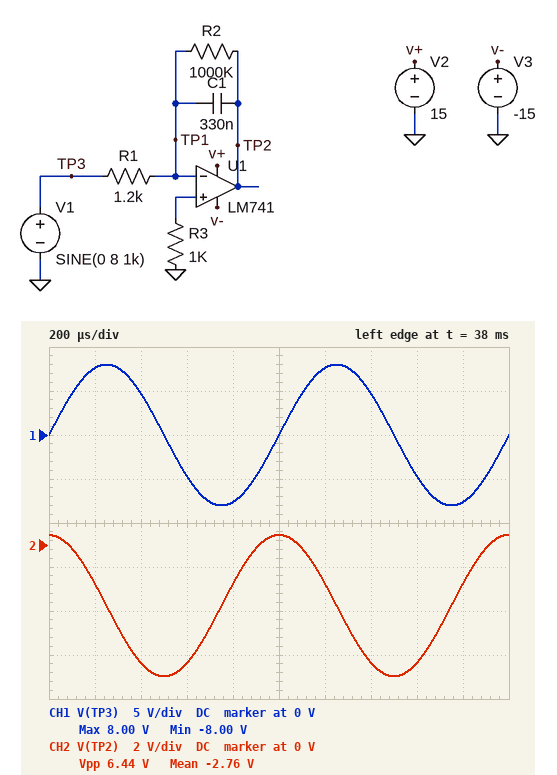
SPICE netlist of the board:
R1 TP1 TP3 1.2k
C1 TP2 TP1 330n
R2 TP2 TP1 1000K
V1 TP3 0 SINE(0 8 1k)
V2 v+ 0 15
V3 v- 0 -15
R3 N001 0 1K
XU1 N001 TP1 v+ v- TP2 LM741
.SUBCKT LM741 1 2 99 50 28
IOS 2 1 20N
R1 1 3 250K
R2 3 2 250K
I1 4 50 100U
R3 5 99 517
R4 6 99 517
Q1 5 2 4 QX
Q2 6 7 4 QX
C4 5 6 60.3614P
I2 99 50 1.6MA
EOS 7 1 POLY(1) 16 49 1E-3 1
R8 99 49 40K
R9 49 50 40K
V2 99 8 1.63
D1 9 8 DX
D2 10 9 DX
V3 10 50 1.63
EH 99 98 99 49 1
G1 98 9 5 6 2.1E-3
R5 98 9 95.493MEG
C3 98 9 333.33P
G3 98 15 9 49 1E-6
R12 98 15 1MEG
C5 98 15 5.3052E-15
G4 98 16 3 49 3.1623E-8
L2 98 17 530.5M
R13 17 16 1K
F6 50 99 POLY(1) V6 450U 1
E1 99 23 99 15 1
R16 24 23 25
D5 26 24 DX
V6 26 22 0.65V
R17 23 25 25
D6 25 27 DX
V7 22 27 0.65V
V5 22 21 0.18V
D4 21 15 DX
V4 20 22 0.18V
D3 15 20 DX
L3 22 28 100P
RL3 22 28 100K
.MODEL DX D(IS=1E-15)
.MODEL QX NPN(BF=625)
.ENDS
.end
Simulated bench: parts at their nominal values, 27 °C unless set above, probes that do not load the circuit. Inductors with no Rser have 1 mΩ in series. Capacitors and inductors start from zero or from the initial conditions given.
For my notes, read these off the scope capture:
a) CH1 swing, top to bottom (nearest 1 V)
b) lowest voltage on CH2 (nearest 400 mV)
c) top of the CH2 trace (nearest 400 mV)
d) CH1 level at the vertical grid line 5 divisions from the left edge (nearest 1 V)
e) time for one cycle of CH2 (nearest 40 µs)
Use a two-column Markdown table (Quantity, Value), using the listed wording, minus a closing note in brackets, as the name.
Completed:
| Quantity | Value |
|---|---|
| CH1 swing, top to bottom | 16 V |
| lowest voltage on CH2 | -6.0 V |
| top of the CH2 trace | 400 mV |
| CH1 level at the vertical grid line 5 divisions from the left edge | 0 V |
| time for one cycle of CH2 | 1.00 ms |
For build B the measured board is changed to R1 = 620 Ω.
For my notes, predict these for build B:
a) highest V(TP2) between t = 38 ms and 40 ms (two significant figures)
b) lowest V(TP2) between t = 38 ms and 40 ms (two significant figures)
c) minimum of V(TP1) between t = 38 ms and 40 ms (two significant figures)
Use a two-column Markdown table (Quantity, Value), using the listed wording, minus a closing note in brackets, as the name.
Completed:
| Quantity | Value |
|---|---|
| highest V(TP2) between t = 38 ms and 40 ms | 900 mV |
| lowest V(TP2) between t = 38 ms and 40 ms | -12 V |
| minimum of V(TP1) between t = 38 ms and 40 ms | -5.3 mV |
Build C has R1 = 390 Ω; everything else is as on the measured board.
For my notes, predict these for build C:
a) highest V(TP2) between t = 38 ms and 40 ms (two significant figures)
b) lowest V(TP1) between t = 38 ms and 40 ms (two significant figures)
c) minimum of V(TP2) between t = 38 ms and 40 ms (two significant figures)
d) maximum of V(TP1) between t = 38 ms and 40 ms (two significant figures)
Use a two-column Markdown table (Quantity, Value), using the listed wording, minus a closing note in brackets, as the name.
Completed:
| Quantity | Value |
|---|---|
| highest V(TP2) between t = 38 ms and 40 ms | 6.4 V |
| lowest V(TP1) between t = 38 ms and 40 ms | -9.3 mV |
| minimum of V(TP2) between t = 38 ms and 40 ms | -13 V |
| maximum of V(TP1) between t = 38 ms and 40 ms | 11 mV |
